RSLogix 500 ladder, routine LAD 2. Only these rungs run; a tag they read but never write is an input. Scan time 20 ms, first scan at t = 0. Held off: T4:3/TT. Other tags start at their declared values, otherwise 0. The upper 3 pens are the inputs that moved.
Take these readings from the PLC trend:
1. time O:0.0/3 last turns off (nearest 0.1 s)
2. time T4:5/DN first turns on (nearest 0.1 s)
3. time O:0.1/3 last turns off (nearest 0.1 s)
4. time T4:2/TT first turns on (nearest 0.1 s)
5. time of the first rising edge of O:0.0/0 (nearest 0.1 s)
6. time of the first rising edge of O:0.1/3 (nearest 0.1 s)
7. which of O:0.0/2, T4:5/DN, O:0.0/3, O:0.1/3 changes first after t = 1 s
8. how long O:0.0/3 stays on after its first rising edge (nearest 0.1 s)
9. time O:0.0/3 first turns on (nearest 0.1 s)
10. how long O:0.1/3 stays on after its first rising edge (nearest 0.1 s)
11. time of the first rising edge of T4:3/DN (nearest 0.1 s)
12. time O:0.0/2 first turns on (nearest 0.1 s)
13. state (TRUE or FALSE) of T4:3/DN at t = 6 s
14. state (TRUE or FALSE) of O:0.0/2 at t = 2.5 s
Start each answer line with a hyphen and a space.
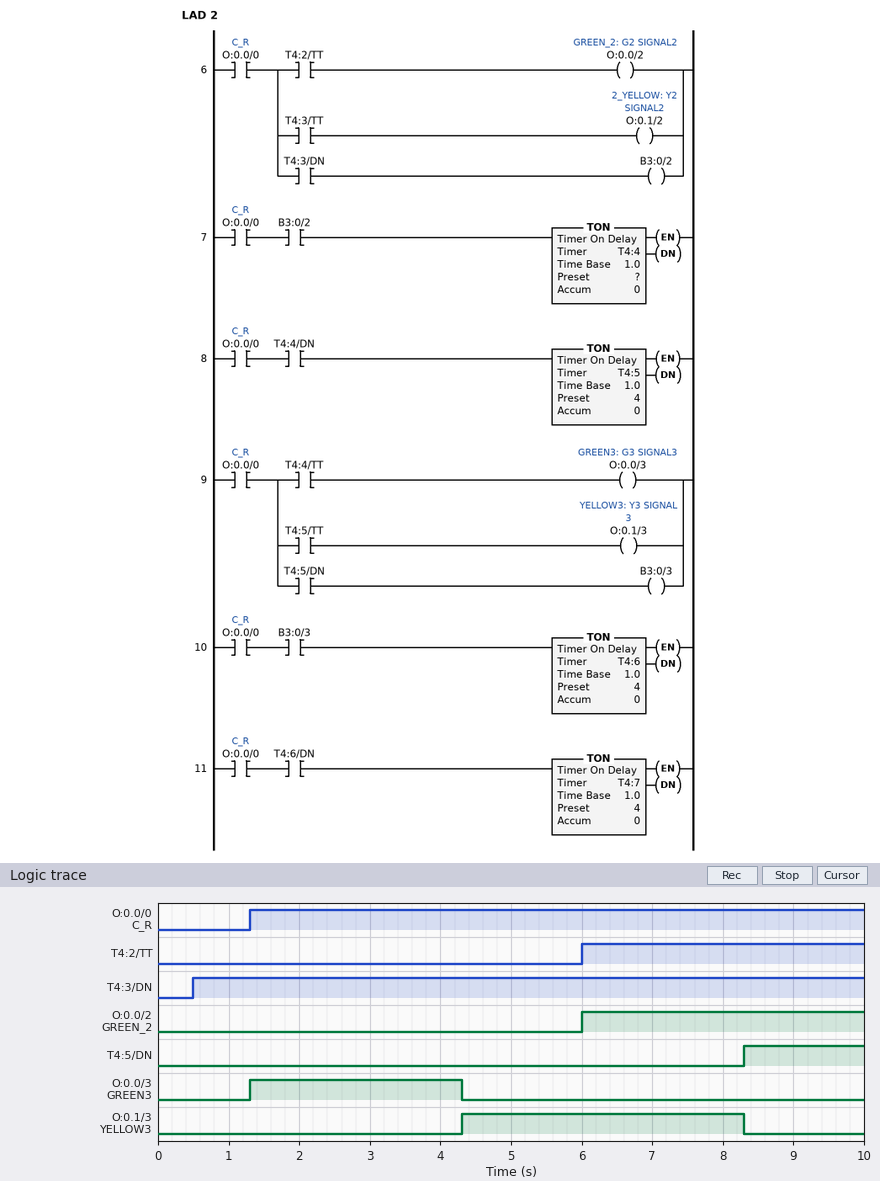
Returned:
- 4.3 s
- 8.3 s
- 8.3 s
- 6.0 s
- 1.3 s
- 4.3 s
- O:0.0/3
- 3.0 s
- 1.3 s
- 4.0 s
- 0.5 s
- 6.0 s
- TRUE
- FALSE
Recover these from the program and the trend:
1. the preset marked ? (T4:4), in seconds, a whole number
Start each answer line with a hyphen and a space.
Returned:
- 3 s
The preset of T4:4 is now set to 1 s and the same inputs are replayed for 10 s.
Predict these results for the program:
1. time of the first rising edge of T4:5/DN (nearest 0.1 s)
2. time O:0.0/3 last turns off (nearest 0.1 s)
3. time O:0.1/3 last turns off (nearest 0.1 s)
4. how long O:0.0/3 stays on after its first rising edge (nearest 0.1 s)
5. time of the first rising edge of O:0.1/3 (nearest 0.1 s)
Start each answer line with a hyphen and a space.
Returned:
- 6.3 s
- 2.3 s
- 6.3 s
- 1.0 s
- 2.3 s
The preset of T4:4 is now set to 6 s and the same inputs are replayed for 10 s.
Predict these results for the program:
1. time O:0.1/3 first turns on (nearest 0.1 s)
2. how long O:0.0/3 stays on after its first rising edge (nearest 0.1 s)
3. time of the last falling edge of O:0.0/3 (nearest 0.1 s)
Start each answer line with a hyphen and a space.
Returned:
- 7.3 s
- 6.0 s
- 7.3 s
